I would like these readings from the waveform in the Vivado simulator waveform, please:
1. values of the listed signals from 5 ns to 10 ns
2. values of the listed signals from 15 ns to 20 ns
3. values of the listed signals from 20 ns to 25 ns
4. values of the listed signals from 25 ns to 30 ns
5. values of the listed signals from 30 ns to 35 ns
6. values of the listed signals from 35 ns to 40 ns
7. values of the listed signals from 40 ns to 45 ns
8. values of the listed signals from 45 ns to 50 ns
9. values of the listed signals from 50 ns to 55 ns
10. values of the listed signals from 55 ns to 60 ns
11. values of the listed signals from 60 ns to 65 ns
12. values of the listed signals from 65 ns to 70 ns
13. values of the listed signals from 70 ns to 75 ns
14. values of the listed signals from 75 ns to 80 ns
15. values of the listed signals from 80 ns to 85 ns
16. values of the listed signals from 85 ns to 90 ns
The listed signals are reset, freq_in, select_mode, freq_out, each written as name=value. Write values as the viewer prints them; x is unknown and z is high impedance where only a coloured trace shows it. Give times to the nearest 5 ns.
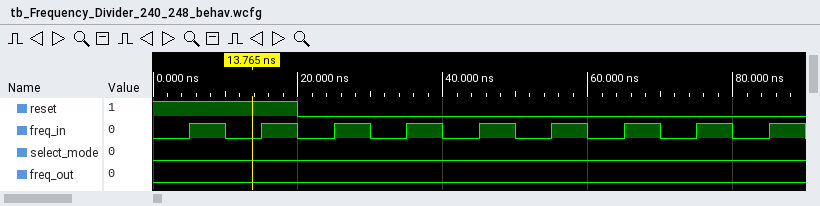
reset=1, freq_in=1, select_mode=0, freq_out=0
reset=1, freq_in=1, select_mode=0, freq_out=0
reset=0, freq_in=0, select_mode=0, freq_out=0
reset=0, freq_in=1, select_mode=0, freq_out=0
reset=0, freq_in=0, select_mode=0, freq_out=0
reset=0, freq_in=1, select_mode=0, freq_out=0
reset=0, freq_in=0, select_mode=0, freq_out=0
reset=0, freq_in=1, select_mode=0, freq_out=0
reset=0, freq_in=0, select_mode=0, freq_out=0
reset=0, freq_in=1, select_mode=0, freq_out=0
reset=0, freq_in=0, select_mode=0, freq_out=0
reset=0, freq_in=1, select_mode=0, freq_out=0
reset=0, freq_in=0, select_mode=0, freq_out=0
reset=0, freq_in=1, select_mode=0, freq_out=0
reset=0, freq_in=0, select_mode=0, freq_out=0
reset=0, freq_in=1, select_mode=0, freq_out=0
